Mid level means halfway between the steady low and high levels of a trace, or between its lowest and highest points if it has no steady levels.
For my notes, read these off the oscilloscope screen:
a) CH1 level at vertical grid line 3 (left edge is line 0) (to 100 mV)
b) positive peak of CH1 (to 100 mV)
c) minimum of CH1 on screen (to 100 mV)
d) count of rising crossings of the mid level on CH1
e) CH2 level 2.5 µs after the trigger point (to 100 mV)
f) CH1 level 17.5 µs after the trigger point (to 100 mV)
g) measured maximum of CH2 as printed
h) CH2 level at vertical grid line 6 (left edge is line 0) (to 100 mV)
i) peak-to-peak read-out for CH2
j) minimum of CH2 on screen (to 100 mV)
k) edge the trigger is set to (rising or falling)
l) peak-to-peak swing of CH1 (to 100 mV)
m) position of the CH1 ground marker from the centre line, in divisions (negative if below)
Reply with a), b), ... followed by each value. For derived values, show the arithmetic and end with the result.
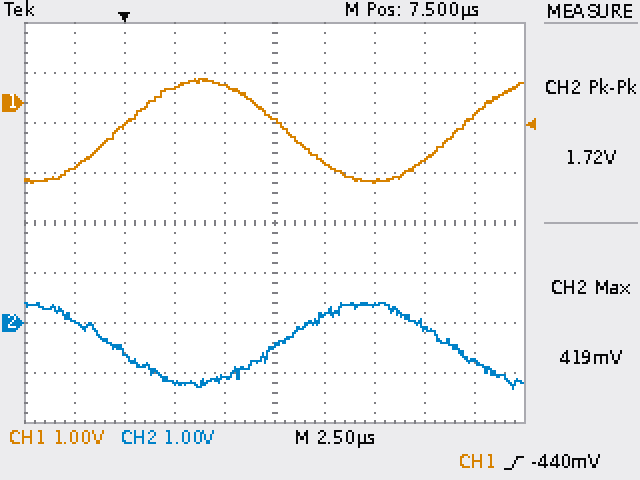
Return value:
a) 300 mV
b) 500 mV
c) -1.6 V
d) 2
e) -1.2 V
f) -200 mV
g) 419 mV
h) 200 mV
i) 1.72 V
j) -1.3 V
k) rising
l) 500 mV − (-1.6 V) = 2.1 V
m) +2.4 div
